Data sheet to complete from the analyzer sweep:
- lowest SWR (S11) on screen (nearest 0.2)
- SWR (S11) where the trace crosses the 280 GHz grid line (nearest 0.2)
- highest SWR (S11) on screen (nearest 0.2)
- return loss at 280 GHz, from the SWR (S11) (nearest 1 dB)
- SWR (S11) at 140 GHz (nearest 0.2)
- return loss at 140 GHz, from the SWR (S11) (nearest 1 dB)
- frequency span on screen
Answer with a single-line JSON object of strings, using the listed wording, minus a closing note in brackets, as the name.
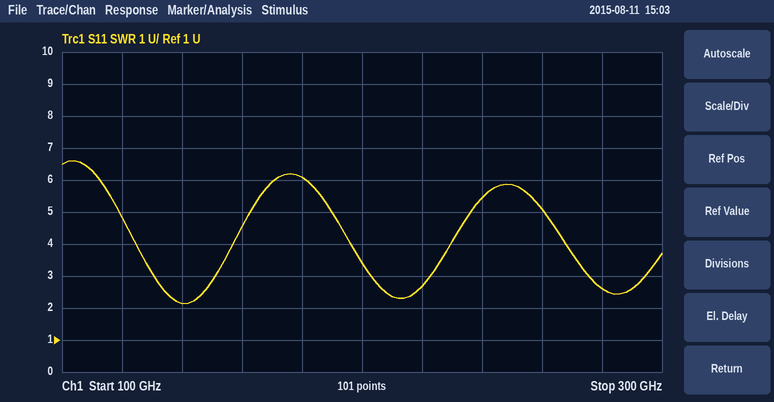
{"lowest SWR (S11) on screen": "2.2", "SWR (S11) where the trace crosses the 280 GHz grid line": "2.6", "highest SWR (S11) on screen": "6.6", "return loss at 280 GHz, from the SWR (S11)": "7 dB", "SWR (S11) at 140 GHz": "2.2", "return loss at 140 GHz, from the SWR (S11)": "9 dB", "frequency span on screen": "200 GHz"}
